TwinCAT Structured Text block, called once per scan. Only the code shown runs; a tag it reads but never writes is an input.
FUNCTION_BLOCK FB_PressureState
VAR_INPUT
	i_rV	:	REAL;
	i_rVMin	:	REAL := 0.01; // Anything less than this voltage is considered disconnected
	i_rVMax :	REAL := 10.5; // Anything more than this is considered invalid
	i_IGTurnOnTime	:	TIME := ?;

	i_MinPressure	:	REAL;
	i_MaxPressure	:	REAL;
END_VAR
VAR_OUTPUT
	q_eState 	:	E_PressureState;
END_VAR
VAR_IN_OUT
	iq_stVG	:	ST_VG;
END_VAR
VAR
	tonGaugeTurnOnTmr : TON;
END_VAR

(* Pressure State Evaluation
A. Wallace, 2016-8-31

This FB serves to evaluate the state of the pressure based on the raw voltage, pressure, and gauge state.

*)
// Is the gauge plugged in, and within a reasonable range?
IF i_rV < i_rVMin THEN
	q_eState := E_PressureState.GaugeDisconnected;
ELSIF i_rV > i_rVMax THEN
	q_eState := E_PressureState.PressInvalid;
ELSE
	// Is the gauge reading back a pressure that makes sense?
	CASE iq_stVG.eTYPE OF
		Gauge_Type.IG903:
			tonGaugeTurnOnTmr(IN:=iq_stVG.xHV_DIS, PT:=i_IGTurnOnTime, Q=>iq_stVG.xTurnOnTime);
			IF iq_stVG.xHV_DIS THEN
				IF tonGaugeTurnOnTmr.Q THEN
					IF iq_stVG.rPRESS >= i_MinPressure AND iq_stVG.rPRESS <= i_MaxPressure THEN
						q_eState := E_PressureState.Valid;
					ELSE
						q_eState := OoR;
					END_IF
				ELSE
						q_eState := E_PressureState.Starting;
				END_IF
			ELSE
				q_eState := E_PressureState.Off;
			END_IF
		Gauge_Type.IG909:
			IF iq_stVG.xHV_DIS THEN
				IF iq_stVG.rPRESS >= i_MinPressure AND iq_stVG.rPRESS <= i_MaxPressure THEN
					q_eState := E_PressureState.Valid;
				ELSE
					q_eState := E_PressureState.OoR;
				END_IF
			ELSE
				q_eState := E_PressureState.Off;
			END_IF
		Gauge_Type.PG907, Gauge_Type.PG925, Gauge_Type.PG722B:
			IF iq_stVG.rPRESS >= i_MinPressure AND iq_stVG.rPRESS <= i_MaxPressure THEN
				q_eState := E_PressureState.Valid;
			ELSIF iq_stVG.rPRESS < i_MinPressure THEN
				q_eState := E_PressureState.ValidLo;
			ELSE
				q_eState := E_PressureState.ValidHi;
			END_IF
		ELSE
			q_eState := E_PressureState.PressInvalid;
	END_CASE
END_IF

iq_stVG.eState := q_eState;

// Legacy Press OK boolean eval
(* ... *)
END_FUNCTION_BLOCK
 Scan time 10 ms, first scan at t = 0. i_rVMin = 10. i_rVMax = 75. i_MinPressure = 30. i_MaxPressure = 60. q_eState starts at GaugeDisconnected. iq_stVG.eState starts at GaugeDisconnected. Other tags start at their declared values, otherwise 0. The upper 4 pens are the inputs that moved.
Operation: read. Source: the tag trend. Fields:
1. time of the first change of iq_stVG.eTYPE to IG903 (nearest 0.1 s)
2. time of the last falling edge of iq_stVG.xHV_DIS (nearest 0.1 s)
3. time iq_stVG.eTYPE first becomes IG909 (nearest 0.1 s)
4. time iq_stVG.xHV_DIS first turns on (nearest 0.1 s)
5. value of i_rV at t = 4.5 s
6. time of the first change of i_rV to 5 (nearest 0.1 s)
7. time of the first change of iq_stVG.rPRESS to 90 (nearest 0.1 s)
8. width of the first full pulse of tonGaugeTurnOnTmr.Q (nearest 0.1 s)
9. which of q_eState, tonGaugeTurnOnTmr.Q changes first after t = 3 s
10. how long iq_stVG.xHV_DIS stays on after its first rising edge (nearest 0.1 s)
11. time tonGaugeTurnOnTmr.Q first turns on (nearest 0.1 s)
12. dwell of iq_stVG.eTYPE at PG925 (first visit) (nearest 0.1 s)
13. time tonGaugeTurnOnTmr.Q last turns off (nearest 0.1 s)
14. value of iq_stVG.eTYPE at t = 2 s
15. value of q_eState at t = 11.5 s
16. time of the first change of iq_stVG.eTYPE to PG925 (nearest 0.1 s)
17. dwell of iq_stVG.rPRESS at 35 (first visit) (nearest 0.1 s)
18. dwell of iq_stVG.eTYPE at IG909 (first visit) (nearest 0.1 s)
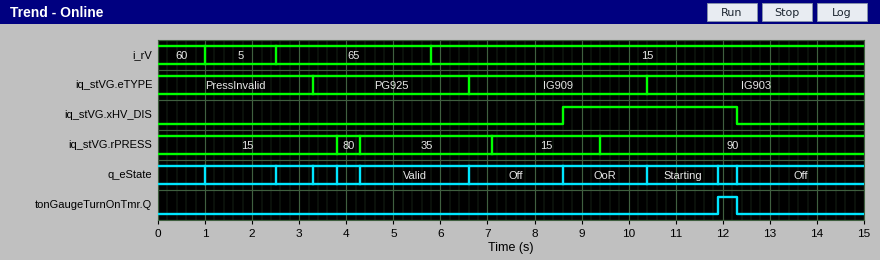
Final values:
10.4 s
12.3 s
6.6 s
8.6 s
65
1.0 s
9.4 s
0.4 s
q_eState
3.7 s
11.9 s
3.3 s
12.3 s
PressInvalid
Starting
3.3 s
2.8 s
3.8 s
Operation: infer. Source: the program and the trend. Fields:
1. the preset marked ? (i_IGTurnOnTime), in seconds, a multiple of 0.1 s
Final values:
1.5 s
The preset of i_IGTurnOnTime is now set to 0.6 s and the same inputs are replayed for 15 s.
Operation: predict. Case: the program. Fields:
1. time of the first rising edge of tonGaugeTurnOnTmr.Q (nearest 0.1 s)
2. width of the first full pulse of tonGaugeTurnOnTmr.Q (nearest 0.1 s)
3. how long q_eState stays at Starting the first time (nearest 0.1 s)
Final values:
11.0 s
1.3 s
0.6 s
